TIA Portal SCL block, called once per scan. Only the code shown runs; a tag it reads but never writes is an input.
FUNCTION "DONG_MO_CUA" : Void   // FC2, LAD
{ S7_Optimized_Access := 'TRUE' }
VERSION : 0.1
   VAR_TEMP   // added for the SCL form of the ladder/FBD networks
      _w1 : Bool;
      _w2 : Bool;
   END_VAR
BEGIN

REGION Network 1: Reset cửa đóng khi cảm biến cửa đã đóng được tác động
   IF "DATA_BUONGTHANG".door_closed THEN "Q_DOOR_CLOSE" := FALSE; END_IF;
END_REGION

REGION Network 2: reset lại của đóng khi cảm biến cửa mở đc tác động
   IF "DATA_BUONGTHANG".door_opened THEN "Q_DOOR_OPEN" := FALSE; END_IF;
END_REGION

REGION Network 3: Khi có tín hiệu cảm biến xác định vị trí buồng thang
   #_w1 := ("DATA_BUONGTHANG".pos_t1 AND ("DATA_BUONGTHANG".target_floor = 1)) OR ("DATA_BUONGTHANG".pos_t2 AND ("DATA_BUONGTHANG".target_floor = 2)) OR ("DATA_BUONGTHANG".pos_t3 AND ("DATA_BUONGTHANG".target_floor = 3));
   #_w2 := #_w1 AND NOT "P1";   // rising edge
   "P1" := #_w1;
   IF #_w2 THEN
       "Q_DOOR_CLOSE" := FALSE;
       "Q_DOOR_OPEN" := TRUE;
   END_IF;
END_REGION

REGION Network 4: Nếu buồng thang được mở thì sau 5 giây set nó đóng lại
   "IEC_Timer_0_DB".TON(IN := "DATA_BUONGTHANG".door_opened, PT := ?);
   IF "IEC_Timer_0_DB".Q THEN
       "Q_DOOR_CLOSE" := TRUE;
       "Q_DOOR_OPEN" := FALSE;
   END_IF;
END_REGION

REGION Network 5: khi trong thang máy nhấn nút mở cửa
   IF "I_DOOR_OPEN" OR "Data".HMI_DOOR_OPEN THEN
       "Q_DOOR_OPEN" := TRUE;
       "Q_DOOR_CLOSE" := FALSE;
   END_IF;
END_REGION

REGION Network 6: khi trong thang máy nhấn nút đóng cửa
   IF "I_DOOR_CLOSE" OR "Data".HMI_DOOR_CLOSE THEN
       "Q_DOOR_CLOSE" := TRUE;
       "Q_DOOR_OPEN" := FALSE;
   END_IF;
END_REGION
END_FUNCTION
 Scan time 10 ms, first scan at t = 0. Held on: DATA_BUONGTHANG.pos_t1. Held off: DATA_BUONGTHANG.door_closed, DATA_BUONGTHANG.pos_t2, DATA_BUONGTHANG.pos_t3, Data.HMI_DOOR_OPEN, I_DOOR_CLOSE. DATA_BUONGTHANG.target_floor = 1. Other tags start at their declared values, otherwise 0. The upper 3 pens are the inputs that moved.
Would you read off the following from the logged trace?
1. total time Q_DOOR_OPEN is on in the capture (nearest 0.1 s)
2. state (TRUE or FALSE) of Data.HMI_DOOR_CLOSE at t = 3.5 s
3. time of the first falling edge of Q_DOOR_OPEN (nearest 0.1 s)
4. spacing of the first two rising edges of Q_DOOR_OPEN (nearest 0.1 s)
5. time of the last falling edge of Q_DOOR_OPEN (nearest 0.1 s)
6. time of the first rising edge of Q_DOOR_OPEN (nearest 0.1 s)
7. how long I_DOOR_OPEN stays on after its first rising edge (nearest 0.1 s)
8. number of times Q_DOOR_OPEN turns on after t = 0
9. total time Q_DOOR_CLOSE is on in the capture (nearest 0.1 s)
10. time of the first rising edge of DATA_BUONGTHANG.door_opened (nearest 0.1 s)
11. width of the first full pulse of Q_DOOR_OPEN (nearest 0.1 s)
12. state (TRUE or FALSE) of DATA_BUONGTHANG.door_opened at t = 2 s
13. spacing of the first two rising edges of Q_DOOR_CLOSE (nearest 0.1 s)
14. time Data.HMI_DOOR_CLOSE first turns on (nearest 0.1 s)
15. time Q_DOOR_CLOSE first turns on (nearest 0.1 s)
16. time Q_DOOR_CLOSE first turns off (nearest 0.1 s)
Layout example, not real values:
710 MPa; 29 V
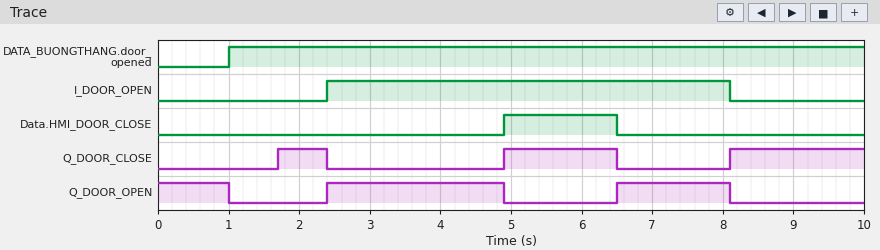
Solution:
5.1 s; FALSE; 1.0 s; 4.1 s; 8.1 s; 2.4 s; 5.7 s; 2; 4.2 s; 1.0 s; 2.5 s; TRUE; 3.2 s; 4.9 s; 1.7 s; 2.4 s
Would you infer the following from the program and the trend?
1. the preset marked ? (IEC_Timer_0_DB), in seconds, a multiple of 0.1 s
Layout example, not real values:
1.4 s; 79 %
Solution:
0.7 s
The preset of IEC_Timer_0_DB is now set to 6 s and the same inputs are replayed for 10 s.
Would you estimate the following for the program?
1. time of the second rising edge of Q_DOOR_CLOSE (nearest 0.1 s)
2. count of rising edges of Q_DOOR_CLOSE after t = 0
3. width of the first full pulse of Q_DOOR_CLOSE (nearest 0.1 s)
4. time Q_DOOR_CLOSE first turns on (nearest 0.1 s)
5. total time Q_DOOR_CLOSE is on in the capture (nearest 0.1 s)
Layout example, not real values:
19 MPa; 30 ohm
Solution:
8.1 s; 2; 1.6 s; 4.9 s; 3.5 s
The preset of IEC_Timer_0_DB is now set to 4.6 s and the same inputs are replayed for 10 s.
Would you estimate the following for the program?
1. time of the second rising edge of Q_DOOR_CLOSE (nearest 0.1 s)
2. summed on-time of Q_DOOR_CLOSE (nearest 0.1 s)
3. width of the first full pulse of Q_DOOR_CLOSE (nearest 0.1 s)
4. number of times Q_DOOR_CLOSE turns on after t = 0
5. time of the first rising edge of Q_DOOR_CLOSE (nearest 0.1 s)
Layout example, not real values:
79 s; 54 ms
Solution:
8.1 s; 3.5 s; 1.6 s; 2; 4.9 s
